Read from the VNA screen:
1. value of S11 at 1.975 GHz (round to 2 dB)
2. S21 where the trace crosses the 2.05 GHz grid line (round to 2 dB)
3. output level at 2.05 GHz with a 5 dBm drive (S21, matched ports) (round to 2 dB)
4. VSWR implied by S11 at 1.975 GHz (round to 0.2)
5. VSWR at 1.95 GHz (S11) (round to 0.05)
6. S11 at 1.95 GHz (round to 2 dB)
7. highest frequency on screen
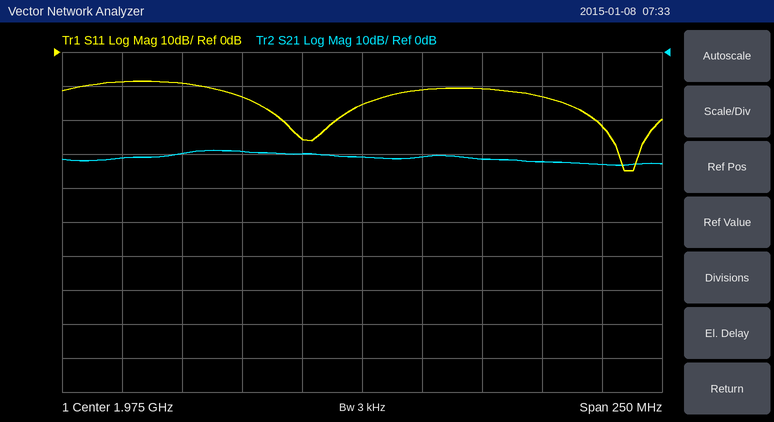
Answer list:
-16 dB
-32 dB
-28 dBm
1.4
1.10
-26 dB
2.1 GHz
